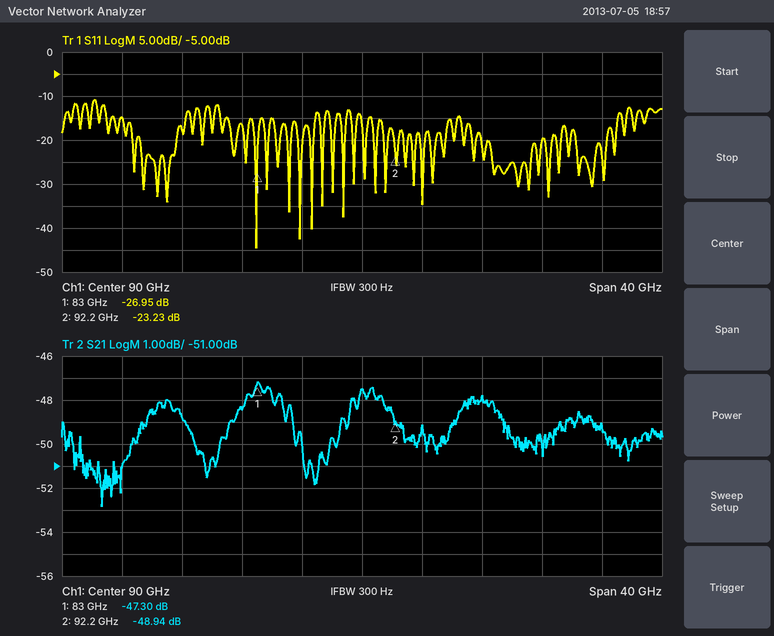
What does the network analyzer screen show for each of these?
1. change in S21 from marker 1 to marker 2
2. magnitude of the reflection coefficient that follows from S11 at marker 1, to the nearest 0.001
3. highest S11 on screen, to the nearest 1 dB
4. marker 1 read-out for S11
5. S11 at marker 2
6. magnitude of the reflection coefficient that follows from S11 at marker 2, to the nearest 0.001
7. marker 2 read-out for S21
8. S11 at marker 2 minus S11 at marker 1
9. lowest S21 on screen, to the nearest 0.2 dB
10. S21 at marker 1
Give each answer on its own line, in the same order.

-1.64 dB
0.045
-11 dB
-26.95 dB
-23.23 dB
0.069
-48.94 dB
3.72 dB
-52.8 dB
-47.30 dB
